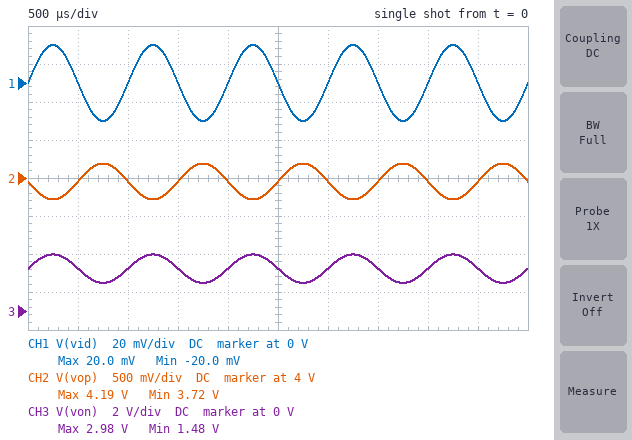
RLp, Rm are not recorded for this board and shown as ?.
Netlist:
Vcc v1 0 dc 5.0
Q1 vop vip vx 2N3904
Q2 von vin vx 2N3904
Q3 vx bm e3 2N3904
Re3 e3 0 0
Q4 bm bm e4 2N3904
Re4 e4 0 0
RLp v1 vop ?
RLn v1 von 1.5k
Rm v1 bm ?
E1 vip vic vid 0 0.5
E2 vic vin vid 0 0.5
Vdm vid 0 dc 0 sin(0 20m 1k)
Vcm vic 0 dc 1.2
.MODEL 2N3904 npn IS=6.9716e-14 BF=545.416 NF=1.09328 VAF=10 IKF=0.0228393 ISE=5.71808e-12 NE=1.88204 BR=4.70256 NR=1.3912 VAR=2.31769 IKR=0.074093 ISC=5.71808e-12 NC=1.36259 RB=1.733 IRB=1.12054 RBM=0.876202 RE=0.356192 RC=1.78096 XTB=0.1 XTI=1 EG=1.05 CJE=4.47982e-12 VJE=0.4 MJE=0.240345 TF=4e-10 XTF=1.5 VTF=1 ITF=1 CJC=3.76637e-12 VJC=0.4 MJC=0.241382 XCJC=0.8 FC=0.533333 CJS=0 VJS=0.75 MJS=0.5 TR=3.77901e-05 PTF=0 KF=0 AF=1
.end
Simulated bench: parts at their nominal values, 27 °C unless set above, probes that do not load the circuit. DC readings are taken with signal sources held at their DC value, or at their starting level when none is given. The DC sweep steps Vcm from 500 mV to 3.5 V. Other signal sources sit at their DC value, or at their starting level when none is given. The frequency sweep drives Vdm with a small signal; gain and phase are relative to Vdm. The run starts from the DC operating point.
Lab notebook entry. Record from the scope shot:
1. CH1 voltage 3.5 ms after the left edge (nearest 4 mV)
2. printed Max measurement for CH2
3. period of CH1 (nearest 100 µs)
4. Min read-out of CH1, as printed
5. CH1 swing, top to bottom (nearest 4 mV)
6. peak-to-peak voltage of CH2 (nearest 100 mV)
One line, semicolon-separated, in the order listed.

0 V; 4.19 V; 1.0 ms; -20.0 mV; 40 mV; 500 mV
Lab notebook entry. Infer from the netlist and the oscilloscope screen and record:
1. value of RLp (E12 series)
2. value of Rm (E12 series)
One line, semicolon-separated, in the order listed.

470 Ω; 1 kΩ
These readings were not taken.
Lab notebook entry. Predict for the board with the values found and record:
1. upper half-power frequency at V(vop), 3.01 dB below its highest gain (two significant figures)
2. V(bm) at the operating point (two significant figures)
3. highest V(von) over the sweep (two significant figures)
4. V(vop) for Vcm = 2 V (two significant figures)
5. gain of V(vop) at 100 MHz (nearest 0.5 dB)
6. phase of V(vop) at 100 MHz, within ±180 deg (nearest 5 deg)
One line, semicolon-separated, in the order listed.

180 MHz; 720 mV; 5.0 V; 3.8 V; 21.0 dB; 145 deg
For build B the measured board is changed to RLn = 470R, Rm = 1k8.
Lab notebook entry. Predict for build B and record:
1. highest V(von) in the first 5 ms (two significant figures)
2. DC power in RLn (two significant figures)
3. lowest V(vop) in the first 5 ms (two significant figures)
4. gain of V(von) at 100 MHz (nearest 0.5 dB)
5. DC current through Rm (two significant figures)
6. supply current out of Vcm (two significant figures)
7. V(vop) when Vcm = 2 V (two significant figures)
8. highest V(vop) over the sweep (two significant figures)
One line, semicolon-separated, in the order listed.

4.6 V; 610 µW; 4.3 V; 17.0 dB; 2.4 mA; 14 µA; 4.4 V; 5.0 V
